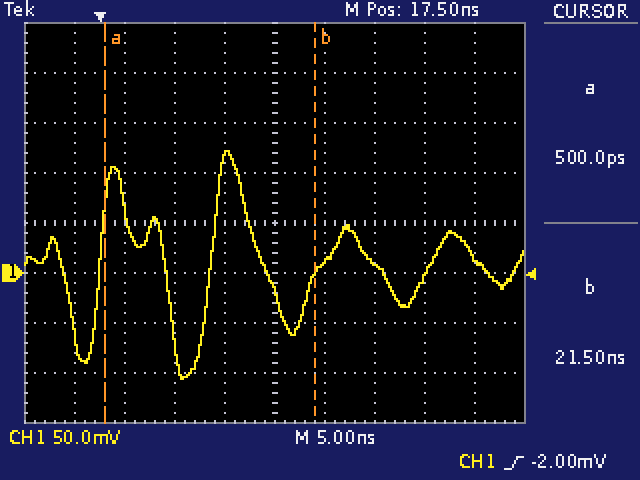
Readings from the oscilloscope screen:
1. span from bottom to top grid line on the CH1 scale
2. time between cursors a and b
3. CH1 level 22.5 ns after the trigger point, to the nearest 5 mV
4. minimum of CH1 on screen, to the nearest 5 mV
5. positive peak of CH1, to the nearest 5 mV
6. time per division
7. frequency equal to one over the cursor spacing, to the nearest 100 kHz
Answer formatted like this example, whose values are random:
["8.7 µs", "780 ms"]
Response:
["400 mV", "21.0 ns", "10 mV", "-105 mV", "120 mV", "5 ns", "47.6 MHz"]
